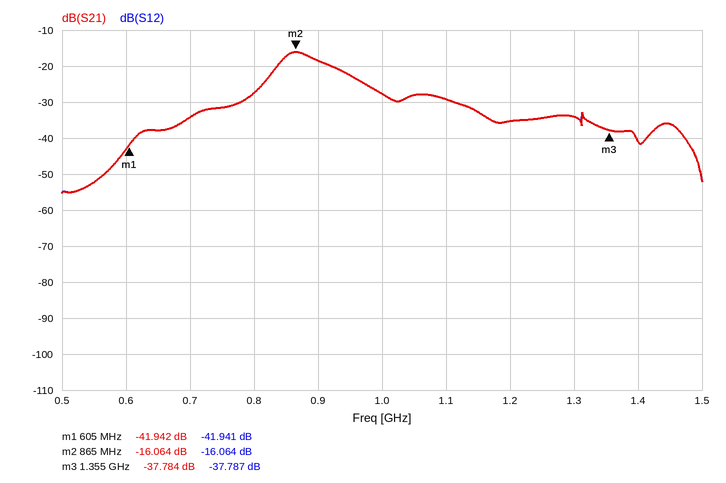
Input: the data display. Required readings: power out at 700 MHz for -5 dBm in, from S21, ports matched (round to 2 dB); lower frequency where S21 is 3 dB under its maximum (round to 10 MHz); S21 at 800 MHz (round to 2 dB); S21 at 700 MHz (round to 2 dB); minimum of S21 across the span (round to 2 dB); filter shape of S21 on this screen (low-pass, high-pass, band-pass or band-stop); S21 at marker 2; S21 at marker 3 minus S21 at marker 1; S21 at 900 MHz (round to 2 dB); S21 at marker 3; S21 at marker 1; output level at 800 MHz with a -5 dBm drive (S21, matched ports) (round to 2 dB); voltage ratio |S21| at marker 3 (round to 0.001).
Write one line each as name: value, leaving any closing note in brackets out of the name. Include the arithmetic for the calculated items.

power out at 700 MHz for -5 dBm in, from S21, ports matched: -5 dBm + (-34 dB) = -40 dBm
lower frequency where S21 is 3 dB under its maximum: 840 MHz
S21 at 800 MHz: -28 dB
S21 at 700 MHz: -34 dB
minimum of S21 across the span: -56 dB
filter shape of S21 on this screen: band-pass
S21 at marker 2: -16.064 dB
S21 at marker 3 minus S21 at marker 1: -37.784 − (-41.942) = 4.158 dB
S21 at 900 MHz: -18 dB
S21 at marker 3: -37.784 dB
S21 at marker 1: -41.942 dB
output level at 800 MHz with a -5 dBm drive (S21, matched ports): -5 dBm + (-28 dB) = -32 dBm
voltage ratio |S21| at marker 3: 10^(-37.784/20) ≈ 0.013
